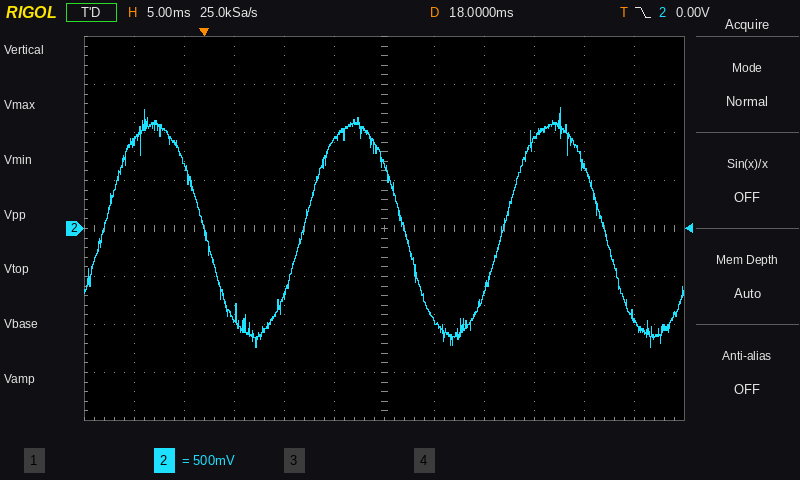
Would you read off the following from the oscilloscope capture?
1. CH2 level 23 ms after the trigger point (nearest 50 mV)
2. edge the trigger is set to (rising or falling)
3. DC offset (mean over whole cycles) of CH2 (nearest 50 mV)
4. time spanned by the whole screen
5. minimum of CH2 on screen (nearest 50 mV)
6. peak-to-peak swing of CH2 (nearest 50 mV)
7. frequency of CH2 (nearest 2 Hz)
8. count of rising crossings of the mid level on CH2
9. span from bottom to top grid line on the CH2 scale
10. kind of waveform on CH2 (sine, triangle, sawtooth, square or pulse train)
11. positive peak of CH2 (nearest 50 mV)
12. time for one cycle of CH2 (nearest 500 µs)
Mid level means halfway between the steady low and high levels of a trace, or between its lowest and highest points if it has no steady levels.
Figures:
-950 mV
falling
0 mV
60 ms
-1.25 V
2.50 V
50 Hz
3
4 V
sine
1.25 V
20.0 ms
